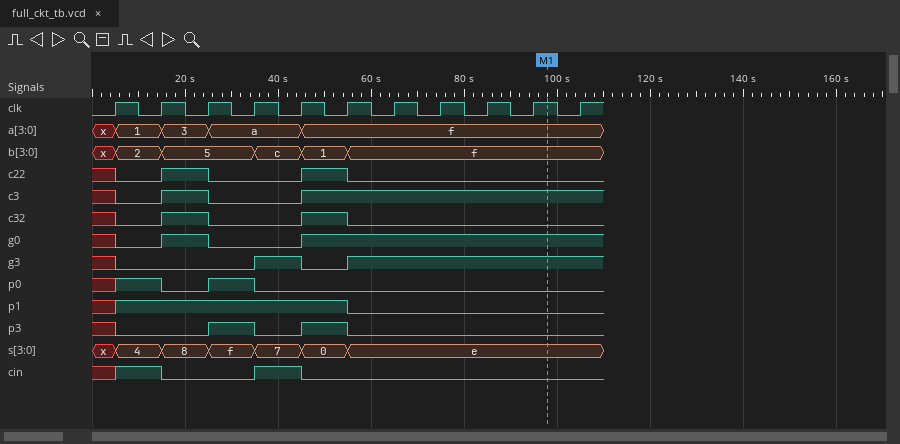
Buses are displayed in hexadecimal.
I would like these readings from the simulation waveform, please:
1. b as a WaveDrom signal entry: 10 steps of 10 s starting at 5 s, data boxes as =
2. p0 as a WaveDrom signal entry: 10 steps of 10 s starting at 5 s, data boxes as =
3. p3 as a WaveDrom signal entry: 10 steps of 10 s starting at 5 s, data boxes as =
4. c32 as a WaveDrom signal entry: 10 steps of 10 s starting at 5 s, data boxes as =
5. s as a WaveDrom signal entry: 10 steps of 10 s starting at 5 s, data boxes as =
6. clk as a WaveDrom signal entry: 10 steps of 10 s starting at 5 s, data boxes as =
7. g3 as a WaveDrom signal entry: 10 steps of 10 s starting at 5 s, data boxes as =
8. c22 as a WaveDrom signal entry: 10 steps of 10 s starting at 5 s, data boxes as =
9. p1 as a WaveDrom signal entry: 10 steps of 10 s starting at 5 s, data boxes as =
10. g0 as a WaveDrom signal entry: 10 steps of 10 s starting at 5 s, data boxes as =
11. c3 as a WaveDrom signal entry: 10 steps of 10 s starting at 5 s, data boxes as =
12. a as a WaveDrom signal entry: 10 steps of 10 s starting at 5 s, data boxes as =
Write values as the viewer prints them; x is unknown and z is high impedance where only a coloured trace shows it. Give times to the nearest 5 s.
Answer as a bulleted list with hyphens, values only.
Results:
- {name: 'b', wave: '==.===....', data: '2 5 c 1 f'}
- {name: 'p0', wave: '1010......'}
- {name: 'p3', wave: '0.1010....'}
- {name: 'c32', wave: '010.10....'}
- {name: 's', wave: '======....', data: '4 8 f 7 0 e'}
- {name: 'clk', wave: 'p.........'}
- {name: 'g3', wave: '0..101....'}
- {name: 'c22', wave: '010.10....'}
- {name: 'p1', wave: '1....0....'}
- {name: 'g0', wave: '010.1.....'}
- {name: 'c3', wave: '010.1.....'}
- {name: 'a', wave: '===.=.....', data: '1 3 a f'}
